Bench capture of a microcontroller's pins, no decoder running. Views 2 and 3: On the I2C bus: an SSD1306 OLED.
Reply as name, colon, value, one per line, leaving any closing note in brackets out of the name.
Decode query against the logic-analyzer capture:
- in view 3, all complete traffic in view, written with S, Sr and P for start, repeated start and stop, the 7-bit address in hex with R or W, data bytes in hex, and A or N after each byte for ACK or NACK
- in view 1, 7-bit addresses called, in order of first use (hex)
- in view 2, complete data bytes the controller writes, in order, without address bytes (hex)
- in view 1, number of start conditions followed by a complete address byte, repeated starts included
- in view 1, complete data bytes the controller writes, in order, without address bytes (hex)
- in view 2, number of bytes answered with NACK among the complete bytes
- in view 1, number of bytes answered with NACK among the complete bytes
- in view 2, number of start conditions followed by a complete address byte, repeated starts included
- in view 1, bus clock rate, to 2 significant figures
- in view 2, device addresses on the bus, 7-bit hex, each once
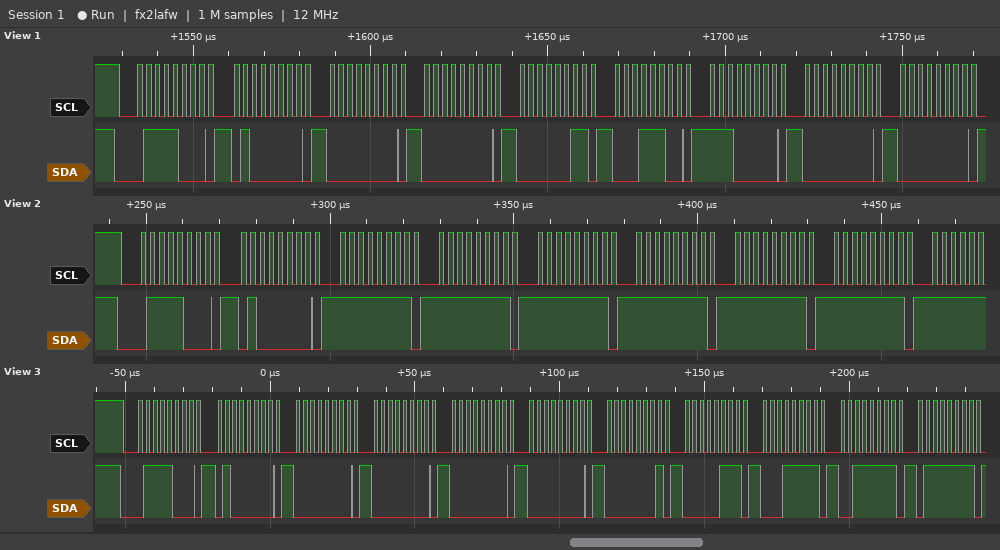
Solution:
in view 3, all complete traffic in view, written with S, Sr and P for start, repeated start and stop, the 7-bit address in hex with R or W, data bytes in hex, and A or N after each byte for ACK or NACK: S 3CW A 40 A 00 A 00 A 00 A 00 A 01 A 07 A 1F A 3F A 7F A
in view 1, 7-bit addresses called, in order of first use: 0x3C
in view 2, complete data bytes the controller writes, in order, without address bytes: 40 FF FF FF FF FF FF
in view 1, number of start conditions followed by a complete address byte, repeated starts included: 1
in view 1, complete data bytes the controller writes, in order, without address bytes: 40 00 00 03 1C E0 00 00
in view 2, number of bytes answered with NACK among the complete bytes: 0
in view 1, number of bytes answered with NACK among the complete bytes: 0
in view 2, number of start conditions followed by a complete address byte, repeated starts included: 1
in view 1, bus clock rate, to 2 significant figures: 400 kHz
in view 2, device addresses on the bus, 7-bit hex, each once: 0x3C
